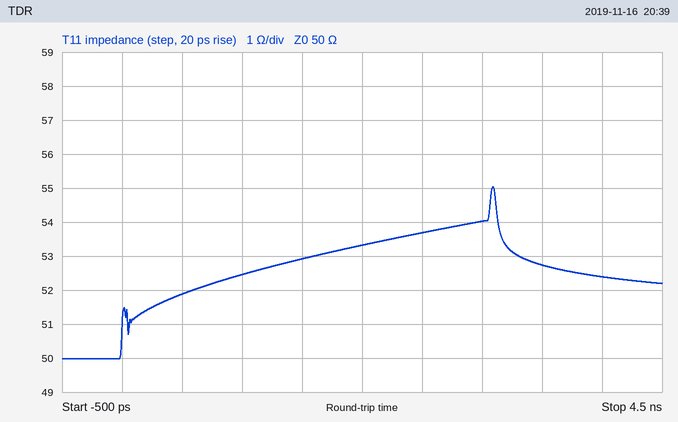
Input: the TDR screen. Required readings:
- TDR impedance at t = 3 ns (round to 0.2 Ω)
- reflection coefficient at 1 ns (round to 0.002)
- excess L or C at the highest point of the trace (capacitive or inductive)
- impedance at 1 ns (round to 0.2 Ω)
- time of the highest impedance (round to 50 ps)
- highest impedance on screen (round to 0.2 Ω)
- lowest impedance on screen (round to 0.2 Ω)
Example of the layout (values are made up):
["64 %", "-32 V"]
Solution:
["54.0 Ω", "+0.024", "inductive", "52.4 Ω", "3.10 ns", "55.0 Ω", "50.0 Ω"]
